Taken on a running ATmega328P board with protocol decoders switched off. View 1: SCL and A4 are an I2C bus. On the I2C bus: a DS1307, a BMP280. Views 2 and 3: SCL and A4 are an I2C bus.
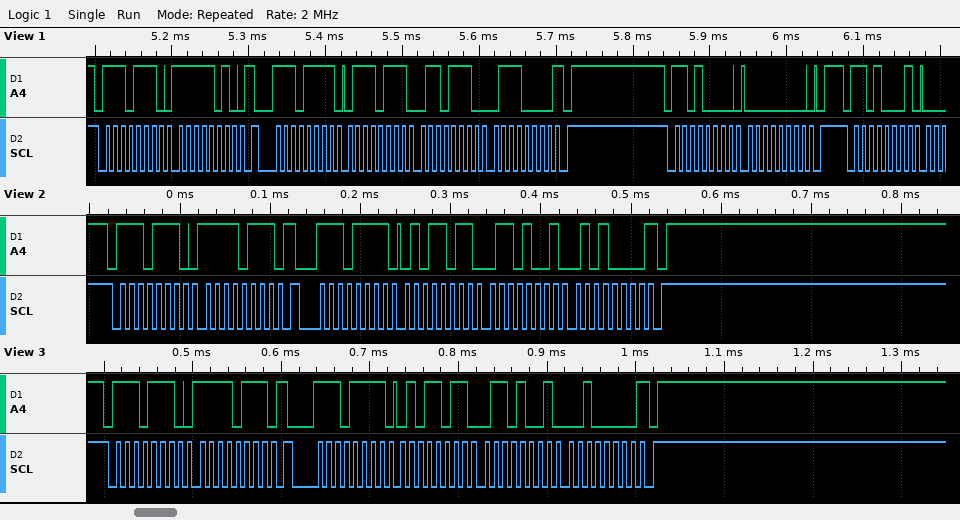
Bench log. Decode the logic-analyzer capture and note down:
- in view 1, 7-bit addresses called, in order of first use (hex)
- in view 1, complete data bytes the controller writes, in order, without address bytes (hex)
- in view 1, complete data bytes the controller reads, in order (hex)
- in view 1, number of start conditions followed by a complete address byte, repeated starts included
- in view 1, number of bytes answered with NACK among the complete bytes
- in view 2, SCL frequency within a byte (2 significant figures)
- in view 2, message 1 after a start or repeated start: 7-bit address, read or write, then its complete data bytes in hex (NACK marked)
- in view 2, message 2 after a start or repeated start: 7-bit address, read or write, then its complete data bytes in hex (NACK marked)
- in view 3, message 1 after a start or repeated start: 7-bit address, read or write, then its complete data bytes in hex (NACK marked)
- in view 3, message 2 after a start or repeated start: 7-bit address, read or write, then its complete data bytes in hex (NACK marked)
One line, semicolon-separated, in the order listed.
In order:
0x77 0x68; FA 00; 77 6E 70; 4; 1; 100 kHz; 0x77 write: F7; 0x77 read: 5B 69 50 NACK; 0x77 write: F7; 0x77 read: 5B 69 20 NACK
